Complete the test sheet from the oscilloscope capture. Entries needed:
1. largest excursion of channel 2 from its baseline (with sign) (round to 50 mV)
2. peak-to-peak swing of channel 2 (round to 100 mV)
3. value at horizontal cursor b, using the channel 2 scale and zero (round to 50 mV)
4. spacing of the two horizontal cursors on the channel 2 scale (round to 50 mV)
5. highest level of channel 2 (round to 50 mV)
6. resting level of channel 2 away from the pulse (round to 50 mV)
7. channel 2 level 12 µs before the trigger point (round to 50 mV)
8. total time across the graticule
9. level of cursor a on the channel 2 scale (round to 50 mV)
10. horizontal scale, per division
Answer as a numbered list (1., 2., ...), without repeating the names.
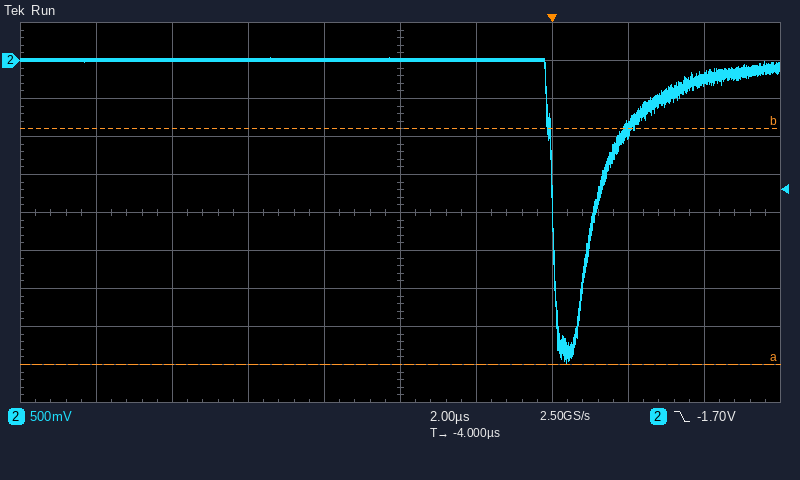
1. -4.00 V
2. 4.00 V
3. -900 mV
4. 3.10 V
5. 50 mV
6. 0 mV
7. 0 mV
8. 20 µs
9. -4.00 V
10. 2 µs
